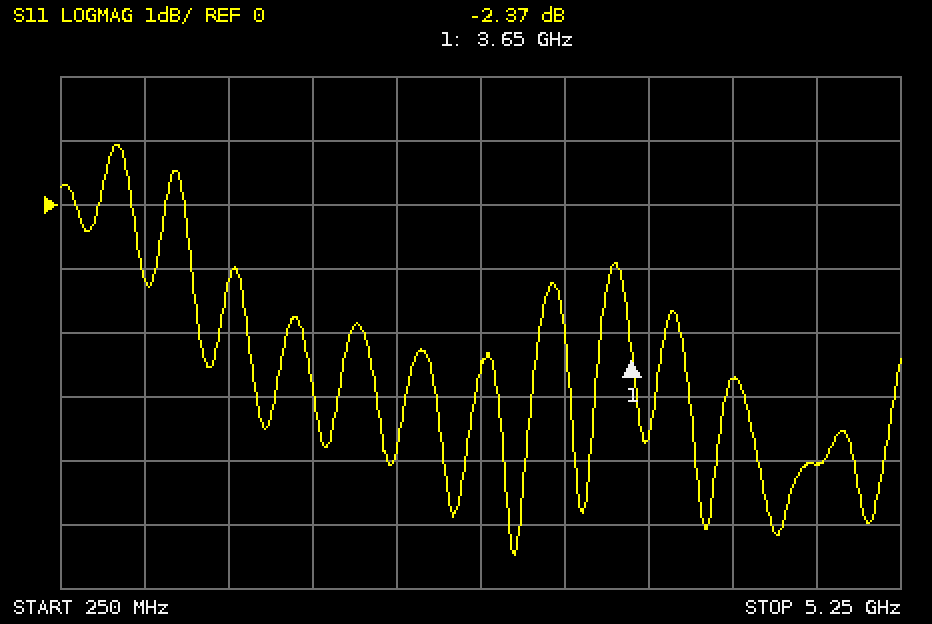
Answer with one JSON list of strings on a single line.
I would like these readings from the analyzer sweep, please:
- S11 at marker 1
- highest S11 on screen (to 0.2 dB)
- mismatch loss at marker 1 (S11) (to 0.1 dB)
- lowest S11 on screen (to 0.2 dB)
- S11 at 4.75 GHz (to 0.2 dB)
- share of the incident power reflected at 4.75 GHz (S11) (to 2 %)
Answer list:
["-2.37 dB", "1.0 dB", "3.8 dB", "-5.4 dB", "-4.0 dB", "40 %"]
